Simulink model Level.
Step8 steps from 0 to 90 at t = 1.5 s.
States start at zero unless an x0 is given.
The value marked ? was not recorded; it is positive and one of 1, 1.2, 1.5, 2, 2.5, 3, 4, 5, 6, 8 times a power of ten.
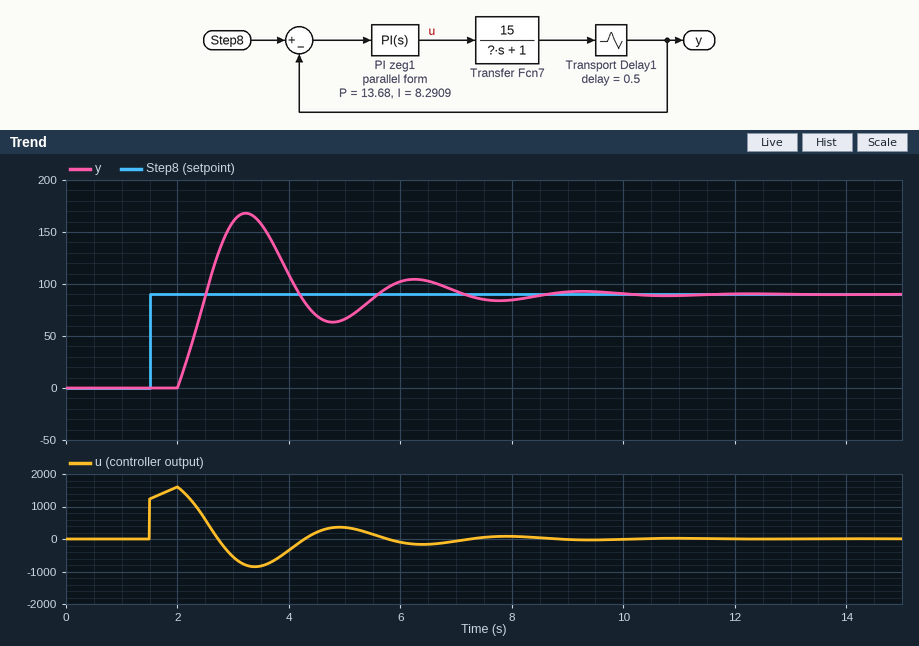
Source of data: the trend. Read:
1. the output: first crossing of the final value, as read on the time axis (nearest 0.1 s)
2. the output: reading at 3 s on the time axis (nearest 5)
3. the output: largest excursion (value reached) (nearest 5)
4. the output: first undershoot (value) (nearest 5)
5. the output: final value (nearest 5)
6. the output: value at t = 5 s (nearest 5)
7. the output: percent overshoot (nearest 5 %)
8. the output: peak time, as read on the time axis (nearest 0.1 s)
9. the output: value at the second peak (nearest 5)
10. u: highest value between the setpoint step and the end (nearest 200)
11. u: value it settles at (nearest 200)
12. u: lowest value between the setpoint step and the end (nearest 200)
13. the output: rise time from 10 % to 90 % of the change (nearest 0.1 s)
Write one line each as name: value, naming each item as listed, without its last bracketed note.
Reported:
the output: first crossing of the final value, as read on the time axis: 2.5 s
the output: reading at 3 s on the time axis: 160
the output: largest excursion (value reached): 170
the output: first undershoot (value): 65
the output: final value: 90
the output: value at t = 5 s: 65
the output: percent overshoot: 85 %
the output: peak time, as read on the time axis: 3.2 s
the output: value at the second peak: 105
u: highest value between the setpoint step and the end: 1600
u: value it settles at: 0
u: lowest value between the setpoint step and the end: -800
the output: rise time from 10 % to 90 % of the change: 0.4 s
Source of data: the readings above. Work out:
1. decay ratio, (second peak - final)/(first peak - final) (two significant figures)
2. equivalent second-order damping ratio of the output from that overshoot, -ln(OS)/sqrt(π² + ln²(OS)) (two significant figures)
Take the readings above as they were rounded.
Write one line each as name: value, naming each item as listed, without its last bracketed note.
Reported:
decay ratio, (second peak - final)/(first peak - final): 0.19
equivalent second-order damping ratio of the output from that overshoot, -ln(OS)/sqrt(π² + ln²(OS)): 0.052
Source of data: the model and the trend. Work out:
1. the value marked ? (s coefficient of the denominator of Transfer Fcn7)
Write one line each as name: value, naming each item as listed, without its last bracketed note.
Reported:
the value marked ?: 120
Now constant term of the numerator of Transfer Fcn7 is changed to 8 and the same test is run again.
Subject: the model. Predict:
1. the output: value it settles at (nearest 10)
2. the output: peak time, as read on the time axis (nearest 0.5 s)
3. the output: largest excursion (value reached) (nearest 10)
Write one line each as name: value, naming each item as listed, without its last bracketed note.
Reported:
the output: value it settles at: 90
the output: peak time, as read on the time axis: 4.0 s
the output: largest excursion (value reached): 140
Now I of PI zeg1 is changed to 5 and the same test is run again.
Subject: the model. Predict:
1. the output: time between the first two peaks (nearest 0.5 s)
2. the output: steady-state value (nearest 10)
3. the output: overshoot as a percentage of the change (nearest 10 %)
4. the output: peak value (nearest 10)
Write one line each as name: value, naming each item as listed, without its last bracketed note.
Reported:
the output: time between the first two peaks: 3.0 s
the output: steady-state value: 90
the output: overshoot as a percentage of the change: 70 %
the output: peak value: 150
